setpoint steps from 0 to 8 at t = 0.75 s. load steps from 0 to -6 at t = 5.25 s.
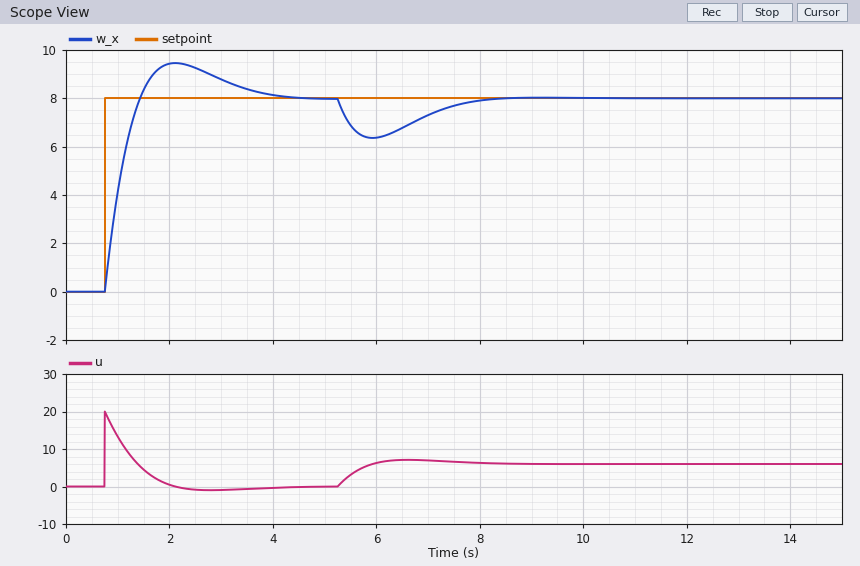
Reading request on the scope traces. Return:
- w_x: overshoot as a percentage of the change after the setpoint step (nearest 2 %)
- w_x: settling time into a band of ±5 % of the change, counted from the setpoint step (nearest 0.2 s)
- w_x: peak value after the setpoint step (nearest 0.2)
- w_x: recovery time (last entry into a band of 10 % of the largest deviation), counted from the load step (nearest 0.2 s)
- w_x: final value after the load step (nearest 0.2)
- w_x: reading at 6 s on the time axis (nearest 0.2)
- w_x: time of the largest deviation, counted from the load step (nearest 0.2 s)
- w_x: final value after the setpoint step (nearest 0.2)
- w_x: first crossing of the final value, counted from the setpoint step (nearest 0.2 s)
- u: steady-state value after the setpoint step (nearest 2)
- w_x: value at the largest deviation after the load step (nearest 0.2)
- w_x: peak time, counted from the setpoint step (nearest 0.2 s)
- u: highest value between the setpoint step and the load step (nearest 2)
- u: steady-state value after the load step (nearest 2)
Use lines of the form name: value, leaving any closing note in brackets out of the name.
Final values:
w_x: overshoot as a percentage of the change after the setpoint step: 18 %
w_x: settling time into a band of ±5 % of the change, counted from the setpoint step: 2.8 s
w_x: peak value after the setpoint step: 9.4
w_x: recovery time (last entry into a band of 10 % of the largest deviation), counted from the load step: 2.6 s
w_x: final value after the load step: 8.0
w_x: reading at 6 s on the time axis: 6.4
w_x: time of the largest deviation, counted from the load step: 0.6 s
w_x: final value after the setpoint step: 8.0
w_x: first crossing of the final value, counted from the setpoint step: 0.6 s
u: steady-state value after the setpoint step: 0
w_x: value at the largest deviation after the load step: 6.4
w_x: peak time, counted from the setpoint step: 1.4 s
u: highest value between the setpoint step and the load step: 20
u: steady-state value after the load step: 6
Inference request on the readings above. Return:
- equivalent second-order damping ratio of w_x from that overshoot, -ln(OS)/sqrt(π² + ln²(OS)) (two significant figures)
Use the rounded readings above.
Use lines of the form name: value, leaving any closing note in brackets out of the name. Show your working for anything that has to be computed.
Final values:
equivalent second-order damping ratio of w_x from that overshoot, -ln(OS)/sqrt(π² + ln²(OS)): ln(0.18) = -1.715; 1.715 / sqrt(9.870 + 2.941) = 0.48
